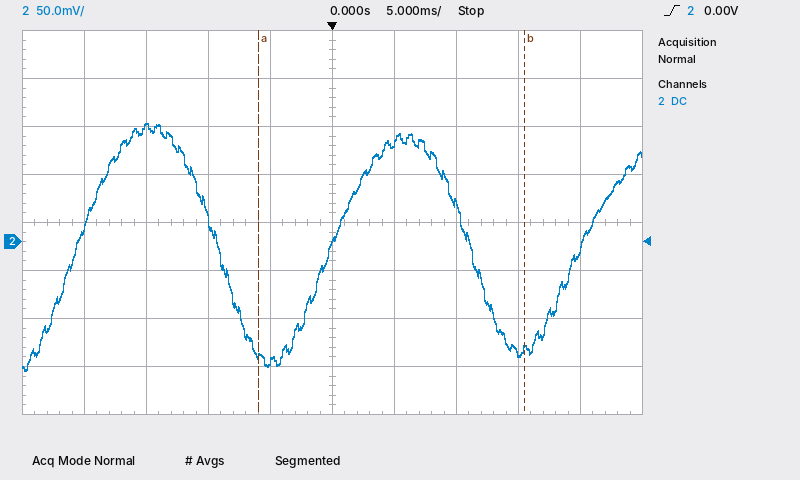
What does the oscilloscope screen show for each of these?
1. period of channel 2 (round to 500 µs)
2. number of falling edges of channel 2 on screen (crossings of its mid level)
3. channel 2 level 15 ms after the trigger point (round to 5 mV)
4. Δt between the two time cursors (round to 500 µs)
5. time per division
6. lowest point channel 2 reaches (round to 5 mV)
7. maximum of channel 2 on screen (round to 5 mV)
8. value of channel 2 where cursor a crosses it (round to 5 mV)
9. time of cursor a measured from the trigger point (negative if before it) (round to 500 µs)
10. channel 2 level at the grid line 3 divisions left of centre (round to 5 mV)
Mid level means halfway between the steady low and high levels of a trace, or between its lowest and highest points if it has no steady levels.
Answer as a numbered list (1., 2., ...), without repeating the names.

1. 20.5 ms
2. 2
3. -115 mV
4. 21.5 ms
5. 5 ms
6. -135 mV
7. 125 mV
8. -120 mV
9. -6.0 ms
10. 120 mV
